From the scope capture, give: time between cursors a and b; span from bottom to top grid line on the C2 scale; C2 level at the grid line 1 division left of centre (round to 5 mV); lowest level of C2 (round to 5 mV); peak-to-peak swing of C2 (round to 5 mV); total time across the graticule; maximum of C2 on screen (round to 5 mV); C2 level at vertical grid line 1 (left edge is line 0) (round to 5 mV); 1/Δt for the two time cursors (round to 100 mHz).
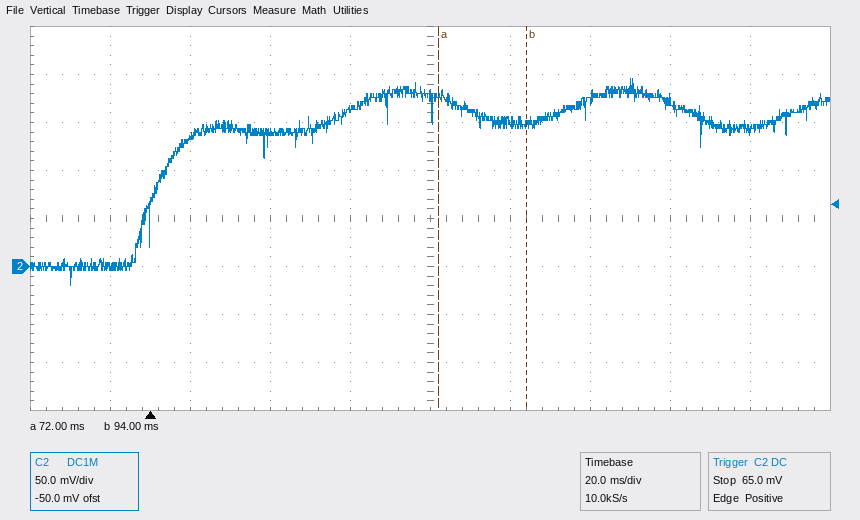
22 ms
400 mV
165 mV
-20 mV
215 mV
200 ms
195 mV
0 mV
45.5 Hz
